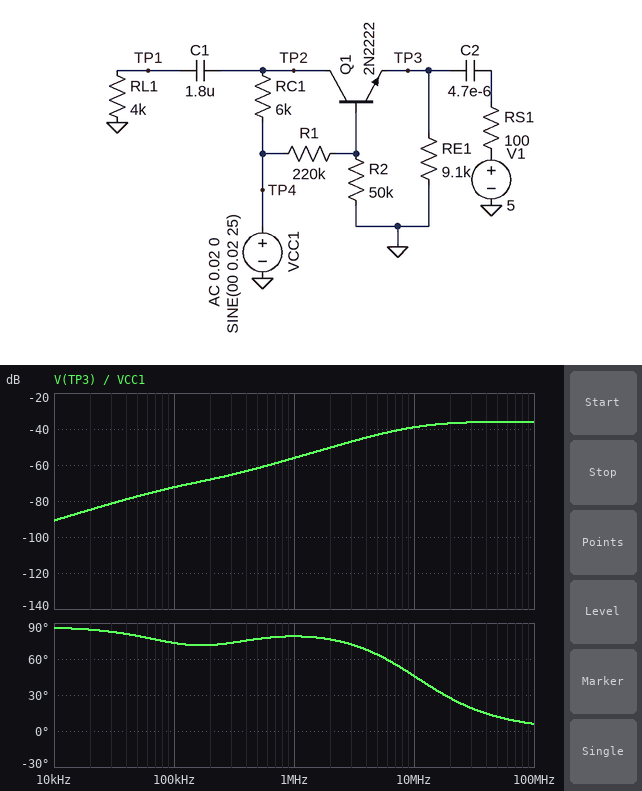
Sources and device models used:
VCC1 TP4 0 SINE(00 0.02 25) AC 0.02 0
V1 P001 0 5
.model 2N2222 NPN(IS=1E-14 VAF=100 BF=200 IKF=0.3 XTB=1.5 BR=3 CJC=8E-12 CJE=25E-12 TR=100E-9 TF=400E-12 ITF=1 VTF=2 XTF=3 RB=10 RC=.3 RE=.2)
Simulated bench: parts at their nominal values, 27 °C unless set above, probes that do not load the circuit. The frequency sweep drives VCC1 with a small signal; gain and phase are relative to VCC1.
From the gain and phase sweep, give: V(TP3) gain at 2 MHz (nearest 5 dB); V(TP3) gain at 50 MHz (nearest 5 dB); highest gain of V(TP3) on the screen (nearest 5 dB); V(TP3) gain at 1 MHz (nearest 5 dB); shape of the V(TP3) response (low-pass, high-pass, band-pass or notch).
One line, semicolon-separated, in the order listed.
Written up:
-50 dB; -35 dB; -35 dB; -55 dB; high-pass
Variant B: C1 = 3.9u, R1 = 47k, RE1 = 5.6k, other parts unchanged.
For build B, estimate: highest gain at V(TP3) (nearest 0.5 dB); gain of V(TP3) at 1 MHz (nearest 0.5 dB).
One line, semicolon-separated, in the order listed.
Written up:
-35.0 dB; -53.0 dB
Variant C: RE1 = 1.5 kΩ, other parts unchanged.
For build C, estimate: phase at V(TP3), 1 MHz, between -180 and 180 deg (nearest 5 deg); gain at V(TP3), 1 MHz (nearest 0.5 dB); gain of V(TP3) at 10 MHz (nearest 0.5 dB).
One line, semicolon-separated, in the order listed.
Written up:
80 deg; -56.5 dB; -39.5 dB
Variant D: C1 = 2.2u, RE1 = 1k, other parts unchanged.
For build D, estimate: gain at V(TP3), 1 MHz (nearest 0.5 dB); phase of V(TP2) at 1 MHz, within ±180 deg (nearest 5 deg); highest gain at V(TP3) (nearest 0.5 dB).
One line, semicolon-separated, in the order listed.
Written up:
-57.0 dB; -5 deg; -36.5 dB
